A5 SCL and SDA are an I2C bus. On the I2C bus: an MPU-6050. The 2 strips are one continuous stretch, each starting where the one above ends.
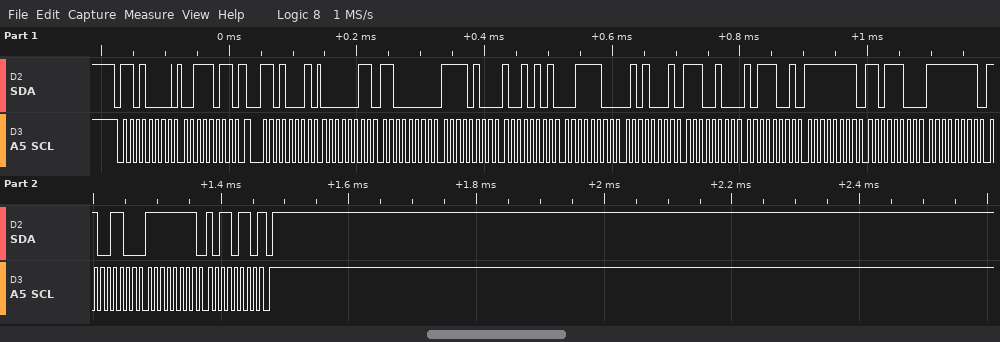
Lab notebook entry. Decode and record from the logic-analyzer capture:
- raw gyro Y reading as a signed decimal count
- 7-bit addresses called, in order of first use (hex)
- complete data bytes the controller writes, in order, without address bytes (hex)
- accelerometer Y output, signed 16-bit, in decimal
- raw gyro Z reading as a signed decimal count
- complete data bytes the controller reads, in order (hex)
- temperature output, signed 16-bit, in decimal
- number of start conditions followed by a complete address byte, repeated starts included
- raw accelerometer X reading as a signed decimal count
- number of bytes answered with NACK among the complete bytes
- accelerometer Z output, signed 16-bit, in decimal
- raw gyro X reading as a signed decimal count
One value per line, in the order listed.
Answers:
-52
0x68
3B
-2923
-74
03 C0 F4 95 3C 51 E4 B9 FF DC FF CC FF B6
-6983
2
960
1
15441
-36
